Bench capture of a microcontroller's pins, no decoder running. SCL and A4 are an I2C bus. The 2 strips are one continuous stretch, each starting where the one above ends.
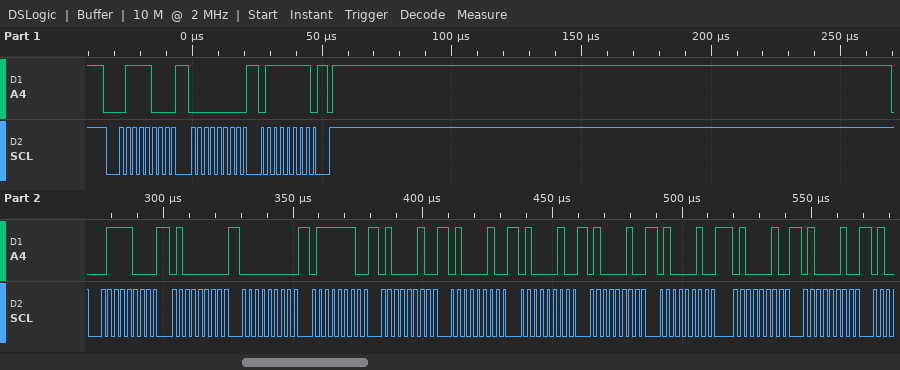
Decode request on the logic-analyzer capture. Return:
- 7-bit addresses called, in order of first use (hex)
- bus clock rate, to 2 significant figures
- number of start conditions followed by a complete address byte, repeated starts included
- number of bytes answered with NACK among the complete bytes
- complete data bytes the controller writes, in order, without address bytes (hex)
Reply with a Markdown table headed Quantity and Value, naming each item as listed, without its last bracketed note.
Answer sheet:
| Quantity | Value |
|---|---|
| 7-bit addresses called, in order of first use | 0x3C |
| bus clock rate, to 2 significant figures | 400 kHz |
| number of start conditions followed by a complete address byte, repeated starts included | 2 |
| number of bytes answered with NACK among the complete bytes | 0 |
| complete data bytes the controller writes, in order, without address bytes | 00 7F 40 00 7E 42 42 42 42 42 42 42 |
